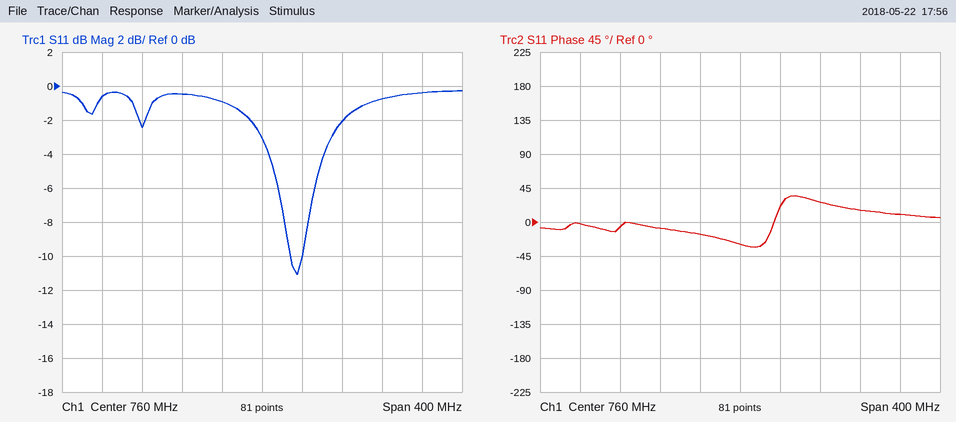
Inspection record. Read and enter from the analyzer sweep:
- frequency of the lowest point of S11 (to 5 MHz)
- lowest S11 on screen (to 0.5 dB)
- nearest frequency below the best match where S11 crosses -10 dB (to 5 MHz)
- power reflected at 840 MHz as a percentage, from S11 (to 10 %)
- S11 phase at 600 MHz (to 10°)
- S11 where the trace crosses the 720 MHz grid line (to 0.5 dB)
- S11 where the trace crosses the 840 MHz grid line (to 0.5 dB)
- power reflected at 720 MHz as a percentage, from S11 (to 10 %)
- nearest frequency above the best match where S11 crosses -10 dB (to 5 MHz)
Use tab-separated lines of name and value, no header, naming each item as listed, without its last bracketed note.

frequency of the lowest point of S11	795 MHz
lowest S11 on screen	-11.0 dB
nearest frequency below the best match where S11 crosses -10 dB	790 MHz
power reflected at 840 MHz as a percentage, from S11	60 %
S11 phase at 600 MHz	0°
S11 where the trace crosses the 720 MHz grid line	-1.0 dB
S11 where the trace crosses the 840 MHz grid line	-2.0 dB
power reflected at 720 MHz as a percentage, from S11	80 %
nearest frequency above the best match where S11 crosses -10 dB	800 MHz
